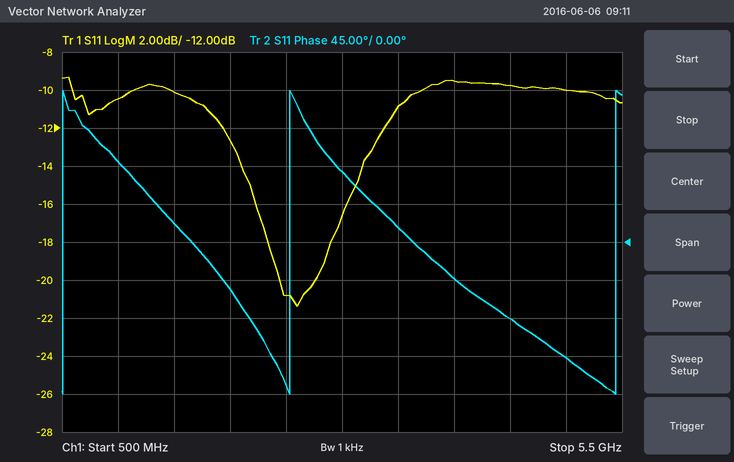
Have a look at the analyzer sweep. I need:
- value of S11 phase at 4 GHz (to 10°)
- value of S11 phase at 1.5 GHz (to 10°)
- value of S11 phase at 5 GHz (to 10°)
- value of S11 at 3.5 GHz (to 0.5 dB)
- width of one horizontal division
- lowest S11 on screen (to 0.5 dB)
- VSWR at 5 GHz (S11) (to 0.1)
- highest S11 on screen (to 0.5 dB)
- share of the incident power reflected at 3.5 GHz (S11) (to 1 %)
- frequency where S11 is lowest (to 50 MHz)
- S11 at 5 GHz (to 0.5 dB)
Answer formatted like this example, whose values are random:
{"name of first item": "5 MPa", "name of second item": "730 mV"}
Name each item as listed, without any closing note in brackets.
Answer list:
{"value of S11 phase at 4 GHz": "-40°", "value of S11 phase at 1.5 GHz": "20°", "value of S11 phase at 5 GHz": "-140°", "value of S11 at 3.5 GHz": "-11.0 dB", "width of one horizontal division": "500 MHz", "lowest S11 on screen": "-21.5 dB", "VSWR at 5 GHz (S11)": "1.9", "highest S11 on screen": "-9.5 dB", "share of the incident power reflected at 3.5 GHz (S11)": "8 %", "frequency where S11 is lowest": "2.60 GHz", "S11 at 5 GHz": "-10.0 dB"}
